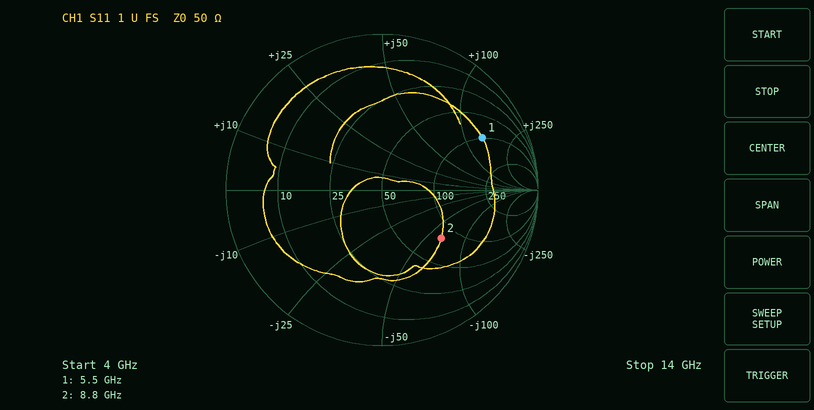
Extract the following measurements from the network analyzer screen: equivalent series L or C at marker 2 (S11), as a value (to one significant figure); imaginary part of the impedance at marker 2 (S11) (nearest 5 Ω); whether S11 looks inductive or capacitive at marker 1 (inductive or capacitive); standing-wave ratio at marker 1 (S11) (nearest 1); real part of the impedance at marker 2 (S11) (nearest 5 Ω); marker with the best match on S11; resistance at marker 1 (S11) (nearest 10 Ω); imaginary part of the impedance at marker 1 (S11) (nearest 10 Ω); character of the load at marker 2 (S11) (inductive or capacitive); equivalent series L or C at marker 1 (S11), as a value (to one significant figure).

300 fF
-65 Ω
inductive
6
80 Ω
marker 2
100 Ω
+140 Ω
capacitive
4 nH
